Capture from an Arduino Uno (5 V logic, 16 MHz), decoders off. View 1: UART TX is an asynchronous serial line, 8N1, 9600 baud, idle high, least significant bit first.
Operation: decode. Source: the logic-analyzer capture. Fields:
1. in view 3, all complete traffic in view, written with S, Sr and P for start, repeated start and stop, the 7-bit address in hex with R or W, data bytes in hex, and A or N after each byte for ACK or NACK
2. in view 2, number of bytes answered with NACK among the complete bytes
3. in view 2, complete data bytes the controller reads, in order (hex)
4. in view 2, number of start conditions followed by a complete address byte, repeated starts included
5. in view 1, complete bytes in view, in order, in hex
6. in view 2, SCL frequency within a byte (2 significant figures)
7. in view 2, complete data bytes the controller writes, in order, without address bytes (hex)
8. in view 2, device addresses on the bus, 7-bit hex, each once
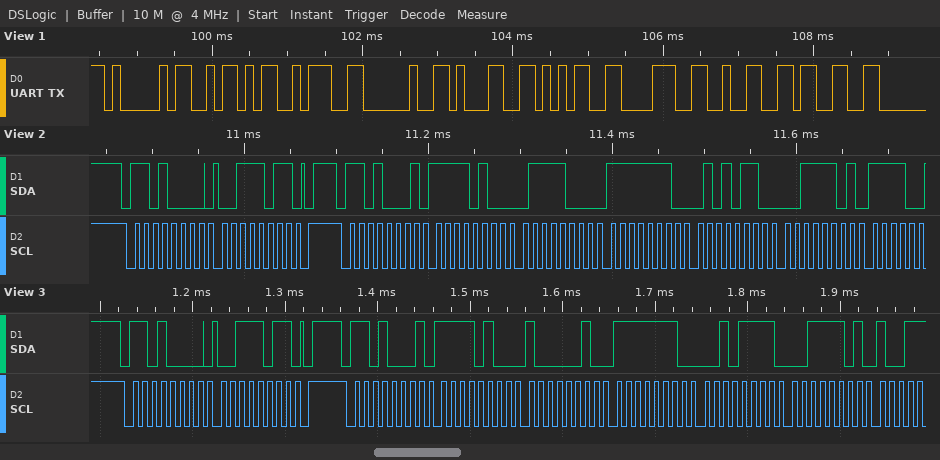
S 68W A 3B A P S 68R A F4 A 82 A FE A 2F A 3D A
0
F4 78 FE 56 3D
2
41 5A 3A 20 31 35 38 32 33
100 kHz
3B
0x68
